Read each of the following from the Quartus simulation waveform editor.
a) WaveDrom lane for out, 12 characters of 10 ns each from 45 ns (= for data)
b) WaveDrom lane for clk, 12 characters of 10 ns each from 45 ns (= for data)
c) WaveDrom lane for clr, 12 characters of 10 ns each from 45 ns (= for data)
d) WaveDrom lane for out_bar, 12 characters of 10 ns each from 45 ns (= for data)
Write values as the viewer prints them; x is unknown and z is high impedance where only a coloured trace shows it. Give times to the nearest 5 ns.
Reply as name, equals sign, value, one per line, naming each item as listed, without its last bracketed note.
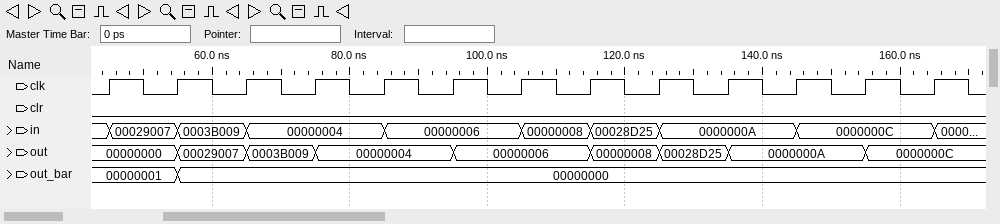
WaveDrom lane for out, 12 characters of 10 ns each from 45 ns = {name: 'out', wave: '====.=.===.=', data: '00000000 00029007 0003B009 00000004 00000006 00000008 00028D25 0000000A 0000000C'}
WaveDrom lane for clk, 12 characters of 10 ns each from 45 ns = {name: 'clk', wave: 'p...........'}
WaveDrom lane for clr, 12 characters of 10 ns each from 45 ns = {name: 'clr', wave: '0...........'}
WaveDrom lane for out_bar, 12 characters of 10 ns each from 45 ns = {name: 'out_bar', wave: '==..........', data: '00000001 00000000'}
